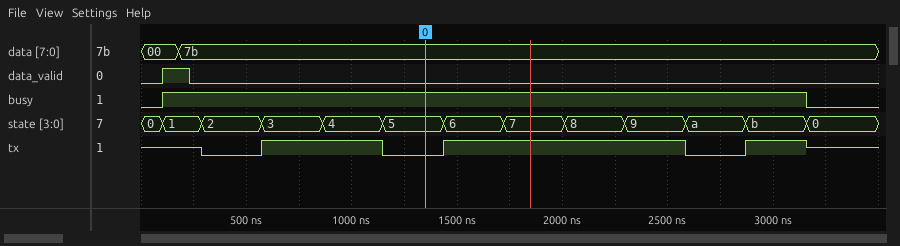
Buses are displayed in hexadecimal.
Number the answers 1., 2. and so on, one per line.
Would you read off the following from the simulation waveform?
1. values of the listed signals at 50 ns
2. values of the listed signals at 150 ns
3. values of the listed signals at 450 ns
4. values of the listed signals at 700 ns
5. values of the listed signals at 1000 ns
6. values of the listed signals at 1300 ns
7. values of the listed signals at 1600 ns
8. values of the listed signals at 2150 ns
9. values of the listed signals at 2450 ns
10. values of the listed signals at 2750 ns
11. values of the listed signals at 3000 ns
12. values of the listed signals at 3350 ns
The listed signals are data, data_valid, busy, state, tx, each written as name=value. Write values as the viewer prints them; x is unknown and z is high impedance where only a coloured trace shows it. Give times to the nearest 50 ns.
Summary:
1. data=00, data_valid=0, busy=0, state=0, tx=z
2. data=00, data_valid=1, busy=1, state=1, tx=z
3. data=7b, data_valid=0, busy=1, state=2, tx=0
4. data=7b, data_valid=0, busy=1, state=3, tx=1
5. data=7b, data_valid=0, busy=1, state=4, tx=1
6. data=7b, data_valid=0, busy=1, state=5, tx=0
7. data=7b, data_valid=0, busy=1, state=6, tx=1
8. data=7b, data_valid=0, busy=1, state=8, tx=1
9. data=7b, data_valid=0, busy=1, state=9, tx=1
10. data=7b, data_valid=0, busy=1, state=a, tx=0
11. data=7b, data_valid=0, busy=1, state=b, tx=1
12. data=7b, data_valid=0, busy=0, state=0, tx=z
